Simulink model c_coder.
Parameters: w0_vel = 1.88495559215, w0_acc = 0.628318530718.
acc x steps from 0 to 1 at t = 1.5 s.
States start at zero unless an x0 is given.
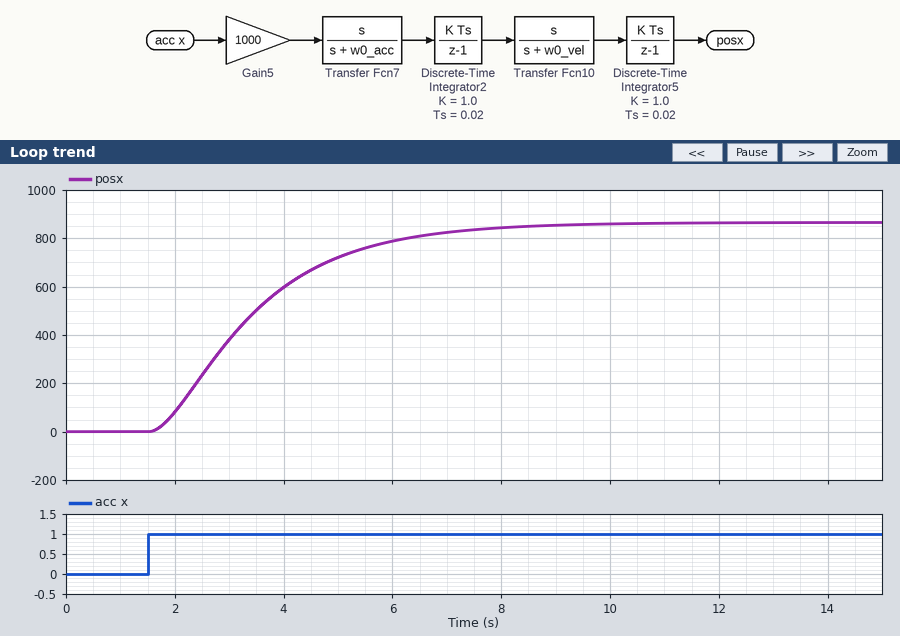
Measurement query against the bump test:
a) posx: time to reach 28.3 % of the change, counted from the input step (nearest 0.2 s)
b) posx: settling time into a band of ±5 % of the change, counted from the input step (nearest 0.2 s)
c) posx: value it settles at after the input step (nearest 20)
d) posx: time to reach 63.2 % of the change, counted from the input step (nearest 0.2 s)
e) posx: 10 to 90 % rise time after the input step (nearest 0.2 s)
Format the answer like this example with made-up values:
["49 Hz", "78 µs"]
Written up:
["1.0 s", "5.4 s", "860", "2.2 s", "3.8 s"]
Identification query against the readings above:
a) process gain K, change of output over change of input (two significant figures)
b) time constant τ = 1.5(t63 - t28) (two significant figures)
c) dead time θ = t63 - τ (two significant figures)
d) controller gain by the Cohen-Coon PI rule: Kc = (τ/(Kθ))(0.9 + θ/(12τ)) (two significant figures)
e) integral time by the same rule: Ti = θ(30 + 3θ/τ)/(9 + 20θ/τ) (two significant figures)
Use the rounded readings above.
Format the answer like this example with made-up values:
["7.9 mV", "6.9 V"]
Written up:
["860", "1.8 s", "0.40 s", "0.0048", "0.91 s"]
